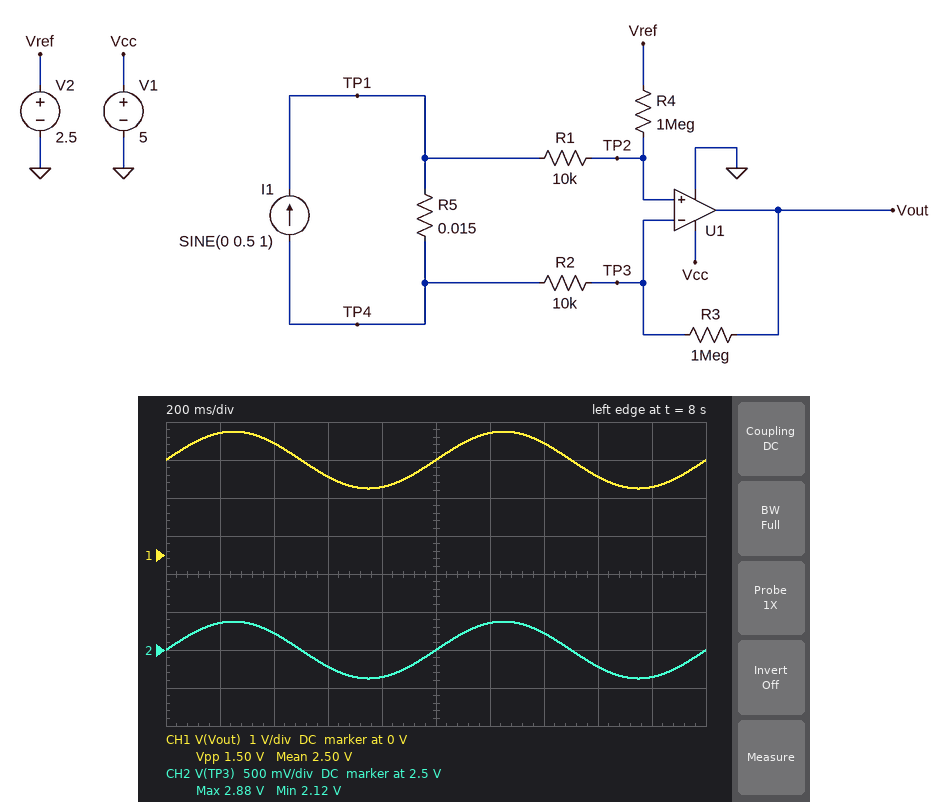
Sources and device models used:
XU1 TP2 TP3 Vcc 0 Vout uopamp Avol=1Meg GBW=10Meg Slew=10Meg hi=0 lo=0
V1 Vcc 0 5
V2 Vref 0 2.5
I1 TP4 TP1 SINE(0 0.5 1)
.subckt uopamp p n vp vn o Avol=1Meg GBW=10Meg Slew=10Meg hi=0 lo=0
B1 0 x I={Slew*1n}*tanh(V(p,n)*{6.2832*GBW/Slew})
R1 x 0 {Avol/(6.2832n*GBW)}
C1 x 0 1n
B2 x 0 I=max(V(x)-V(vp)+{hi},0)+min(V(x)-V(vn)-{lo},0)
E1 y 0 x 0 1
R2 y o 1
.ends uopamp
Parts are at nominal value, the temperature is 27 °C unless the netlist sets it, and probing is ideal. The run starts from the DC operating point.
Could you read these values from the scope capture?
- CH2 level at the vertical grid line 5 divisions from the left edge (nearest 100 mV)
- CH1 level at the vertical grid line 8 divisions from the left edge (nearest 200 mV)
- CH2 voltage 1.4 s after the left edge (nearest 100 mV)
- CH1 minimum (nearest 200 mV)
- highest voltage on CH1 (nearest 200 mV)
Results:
2.5 V
2.0 V
2.7 V
1.8 V
3.2 V
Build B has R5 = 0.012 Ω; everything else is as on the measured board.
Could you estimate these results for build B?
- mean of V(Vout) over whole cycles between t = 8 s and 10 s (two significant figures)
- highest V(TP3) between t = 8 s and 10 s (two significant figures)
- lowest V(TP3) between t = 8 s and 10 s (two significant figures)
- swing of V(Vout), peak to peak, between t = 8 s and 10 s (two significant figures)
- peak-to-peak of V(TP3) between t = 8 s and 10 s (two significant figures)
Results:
2.5 V
2.8 V
2.2 V
1.2 V
600 mV
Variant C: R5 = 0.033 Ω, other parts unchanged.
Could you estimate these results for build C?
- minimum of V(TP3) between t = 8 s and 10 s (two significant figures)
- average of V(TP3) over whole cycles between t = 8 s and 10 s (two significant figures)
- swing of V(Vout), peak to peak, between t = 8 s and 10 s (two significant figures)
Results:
1.7 V
2.5 V
3.3 V
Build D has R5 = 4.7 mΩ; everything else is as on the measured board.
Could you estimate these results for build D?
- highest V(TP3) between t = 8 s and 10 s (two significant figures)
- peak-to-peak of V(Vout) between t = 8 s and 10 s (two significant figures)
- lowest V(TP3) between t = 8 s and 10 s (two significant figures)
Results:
2.6 V
470 mV
2.4 V
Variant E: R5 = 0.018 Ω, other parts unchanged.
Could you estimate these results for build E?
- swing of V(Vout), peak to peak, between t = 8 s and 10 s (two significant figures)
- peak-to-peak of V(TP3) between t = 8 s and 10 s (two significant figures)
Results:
1.8 V
900 mV
